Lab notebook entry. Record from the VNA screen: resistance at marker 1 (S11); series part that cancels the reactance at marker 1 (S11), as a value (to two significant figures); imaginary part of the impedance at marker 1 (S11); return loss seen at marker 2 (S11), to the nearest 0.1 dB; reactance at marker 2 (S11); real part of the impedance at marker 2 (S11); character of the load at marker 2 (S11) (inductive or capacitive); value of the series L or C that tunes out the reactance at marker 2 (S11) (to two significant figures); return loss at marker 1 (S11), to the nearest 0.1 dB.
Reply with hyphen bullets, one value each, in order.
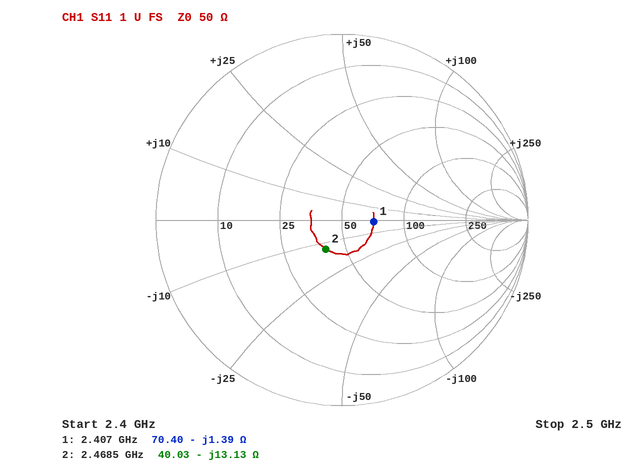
- 70.40 Ω
- 92 pH
- -1.39 Ω
- 14.8 dB
- -13.13 Ω
- 40.03 Ω
- capacitive
- 850 pH
- 15.4 dB
